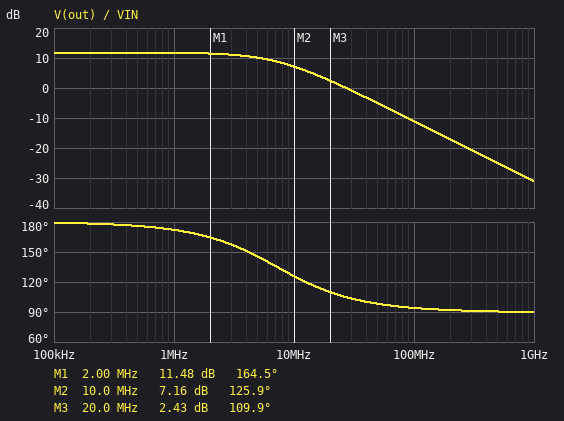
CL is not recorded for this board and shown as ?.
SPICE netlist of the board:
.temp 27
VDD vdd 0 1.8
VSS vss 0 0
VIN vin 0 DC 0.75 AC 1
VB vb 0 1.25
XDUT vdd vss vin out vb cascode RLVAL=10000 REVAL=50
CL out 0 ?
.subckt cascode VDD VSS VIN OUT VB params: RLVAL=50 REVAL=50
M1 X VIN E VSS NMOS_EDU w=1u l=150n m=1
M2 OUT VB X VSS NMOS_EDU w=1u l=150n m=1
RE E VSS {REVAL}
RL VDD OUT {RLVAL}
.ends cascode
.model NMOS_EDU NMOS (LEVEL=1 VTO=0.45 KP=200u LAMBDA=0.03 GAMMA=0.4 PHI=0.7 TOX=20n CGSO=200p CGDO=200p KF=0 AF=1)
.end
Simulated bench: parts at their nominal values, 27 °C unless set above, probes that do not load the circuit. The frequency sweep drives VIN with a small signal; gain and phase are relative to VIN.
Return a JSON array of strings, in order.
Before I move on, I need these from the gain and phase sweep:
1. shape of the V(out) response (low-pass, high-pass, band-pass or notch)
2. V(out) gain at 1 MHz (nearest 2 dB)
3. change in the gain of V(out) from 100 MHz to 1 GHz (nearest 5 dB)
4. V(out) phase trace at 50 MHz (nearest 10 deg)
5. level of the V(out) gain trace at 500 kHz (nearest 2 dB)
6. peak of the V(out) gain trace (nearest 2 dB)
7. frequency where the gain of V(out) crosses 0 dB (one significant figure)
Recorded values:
["low-pass", "12 dB", "-20 dB", "100 deg", "12 dB", "12 dB", "30 MHz"]
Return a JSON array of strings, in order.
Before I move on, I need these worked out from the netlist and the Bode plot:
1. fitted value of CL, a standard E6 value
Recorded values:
["2.2 pF"]
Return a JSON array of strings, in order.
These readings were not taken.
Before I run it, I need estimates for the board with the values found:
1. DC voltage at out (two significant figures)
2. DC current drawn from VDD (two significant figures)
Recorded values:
["1.2 V", "59 µA"]
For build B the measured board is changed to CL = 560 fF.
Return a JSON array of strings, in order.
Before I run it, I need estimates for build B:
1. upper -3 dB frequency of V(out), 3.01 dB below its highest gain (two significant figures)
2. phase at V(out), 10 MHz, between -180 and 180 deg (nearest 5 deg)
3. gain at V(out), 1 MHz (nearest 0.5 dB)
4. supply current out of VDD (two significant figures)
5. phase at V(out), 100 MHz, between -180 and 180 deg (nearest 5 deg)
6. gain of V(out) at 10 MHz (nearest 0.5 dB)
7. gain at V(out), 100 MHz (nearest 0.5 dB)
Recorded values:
["28 MHz", "160 deg", "12.0 dB", "59 µA", "105 deg", "11.5 dB", "0.5 dB"]
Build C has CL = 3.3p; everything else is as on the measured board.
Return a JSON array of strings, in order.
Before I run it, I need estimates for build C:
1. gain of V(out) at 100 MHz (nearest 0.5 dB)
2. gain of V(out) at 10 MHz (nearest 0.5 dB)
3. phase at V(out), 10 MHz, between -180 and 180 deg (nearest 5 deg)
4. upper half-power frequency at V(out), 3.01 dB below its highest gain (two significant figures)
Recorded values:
["-14.5 dB", "4.5 dB", "115 deg", "4.8 MHz"]
